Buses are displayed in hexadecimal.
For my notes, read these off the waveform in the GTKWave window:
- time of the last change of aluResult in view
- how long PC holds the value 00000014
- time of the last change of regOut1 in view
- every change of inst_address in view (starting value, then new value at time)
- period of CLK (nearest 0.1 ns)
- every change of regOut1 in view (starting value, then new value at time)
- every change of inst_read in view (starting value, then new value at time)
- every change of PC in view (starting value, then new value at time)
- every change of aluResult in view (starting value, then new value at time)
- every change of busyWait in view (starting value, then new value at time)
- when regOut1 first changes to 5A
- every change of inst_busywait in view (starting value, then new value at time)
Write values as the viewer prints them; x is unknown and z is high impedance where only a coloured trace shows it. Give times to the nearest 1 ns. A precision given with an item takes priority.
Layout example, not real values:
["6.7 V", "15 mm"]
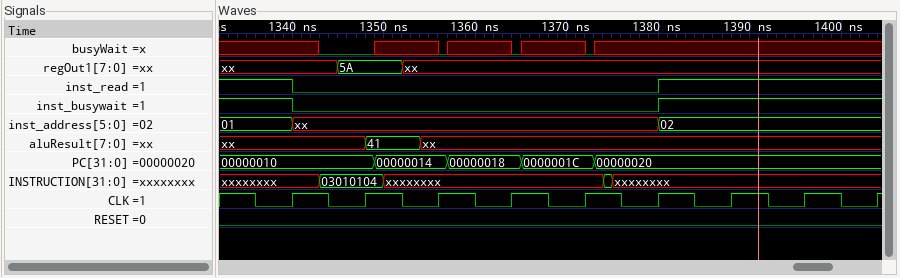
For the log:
["1354 ns", "8 ns", "1352 ns", "01, xx at 1340 ns, 02 at 1380 ns", "8 ns", "xx, 5A at 1345 ns, xx at 1352 ns", "1, 0 at 1340 ns, 1 at 1380 ns", "00000010, 00000014 at 1349 ns, 00000018 at 1357 ns, 0000001C at 1365 ns, 00000020 at 1373 ns", "xx, 41 at 1348 ns, xx at 1354 ns", "x, 0 at 1343 ns, x at 1349 ns, 0 at 1356 ns, x at 1357 ns, 0 at 1364 ns, x at 1365 ns, 0 at 1372 ns, x at 1373 ns", "1345 ns", "1, 0 at 1340 ns, 1 at 1380 ns"]
